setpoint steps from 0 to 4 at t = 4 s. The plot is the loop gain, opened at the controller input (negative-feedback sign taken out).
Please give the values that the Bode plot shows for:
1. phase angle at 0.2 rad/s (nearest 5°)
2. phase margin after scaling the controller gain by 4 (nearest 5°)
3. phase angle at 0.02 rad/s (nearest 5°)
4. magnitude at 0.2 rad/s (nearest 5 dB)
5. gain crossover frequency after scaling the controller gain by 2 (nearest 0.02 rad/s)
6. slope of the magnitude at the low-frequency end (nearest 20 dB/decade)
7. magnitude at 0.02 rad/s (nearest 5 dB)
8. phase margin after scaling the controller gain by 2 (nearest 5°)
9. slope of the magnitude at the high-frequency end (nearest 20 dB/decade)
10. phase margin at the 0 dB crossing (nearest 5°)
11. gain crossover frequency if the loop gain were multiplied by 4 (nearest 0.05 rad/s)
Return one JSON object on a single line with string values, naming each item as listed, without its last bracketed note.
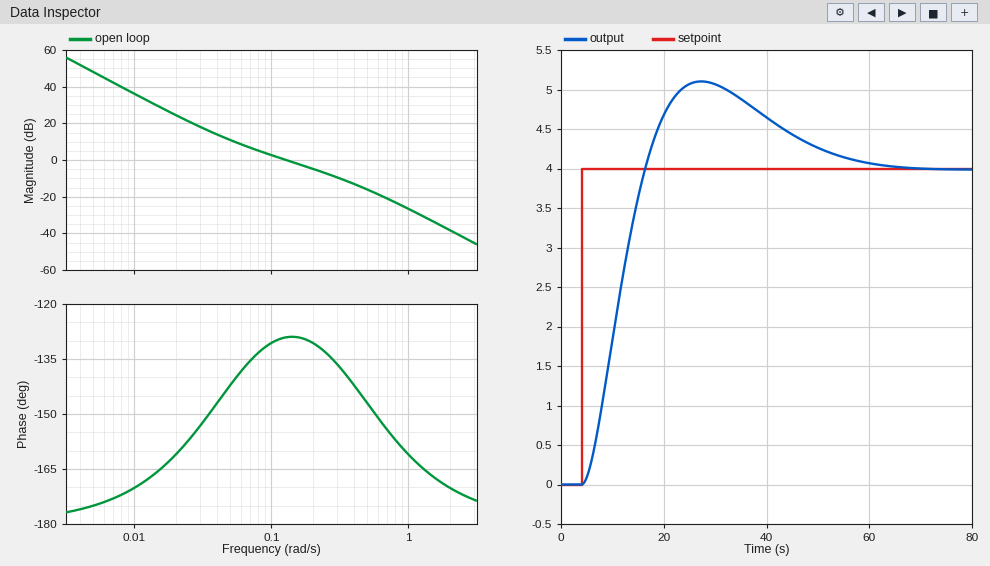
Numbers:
{"phase angle at 0.2 rad/s": "-130°", "phase margin after scaling the controller gain by 4": "40°", "phase angle at 0.02 rad/s": "-160°", "magnitude at 0.2 rad/s": "-5 dB", "gain crossover frequency after scaling the controller gain by 2": "0.22 rad/s", "slope of the magnitude at the low-frequency end": "-40 dB/decade", "magnitude at 0.02 rad/s": "25 dB", "phase margin after scaling the controller gain by 2": "50°", "slope of the magnitude at the high-frequency end": "-40 dB/decade", "phase margin at the 0 dB crossing": "50°", "gain crossover frequency if the loop gain were multiplied by 4": "0.35 rad/s"}
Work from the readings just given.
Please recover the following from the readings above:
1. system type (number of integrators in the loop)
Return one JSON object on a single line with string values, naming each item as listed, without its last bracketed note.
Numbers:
{"system type": "2"}
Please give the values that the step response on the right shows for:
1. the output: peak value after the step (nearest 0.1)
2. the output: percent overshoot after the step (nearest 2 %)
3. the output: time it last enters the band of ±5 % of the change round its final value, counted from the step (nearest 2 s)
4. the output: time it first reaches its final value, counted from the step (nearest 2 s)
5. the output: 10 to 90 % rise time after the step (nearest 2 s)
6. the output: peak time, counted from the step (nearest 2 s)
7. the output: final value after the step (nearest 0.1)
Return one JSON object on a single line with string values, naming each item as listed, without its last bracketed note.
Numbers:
{"the output: peak value after the step": "5.1", "the output: percent overshoot after the step": "28 %", "the output: time it last enters the band of ±5 % of the change round its final value, counted from the step": "48 s", "the output: time it first reaches its final value, counted from the step": "12 s", "the output: 10 to 90 % rise time after the step": "8 s", "the output: peak time, counted from the step": "24 s", "the output: final value after the step": "4.0"}
